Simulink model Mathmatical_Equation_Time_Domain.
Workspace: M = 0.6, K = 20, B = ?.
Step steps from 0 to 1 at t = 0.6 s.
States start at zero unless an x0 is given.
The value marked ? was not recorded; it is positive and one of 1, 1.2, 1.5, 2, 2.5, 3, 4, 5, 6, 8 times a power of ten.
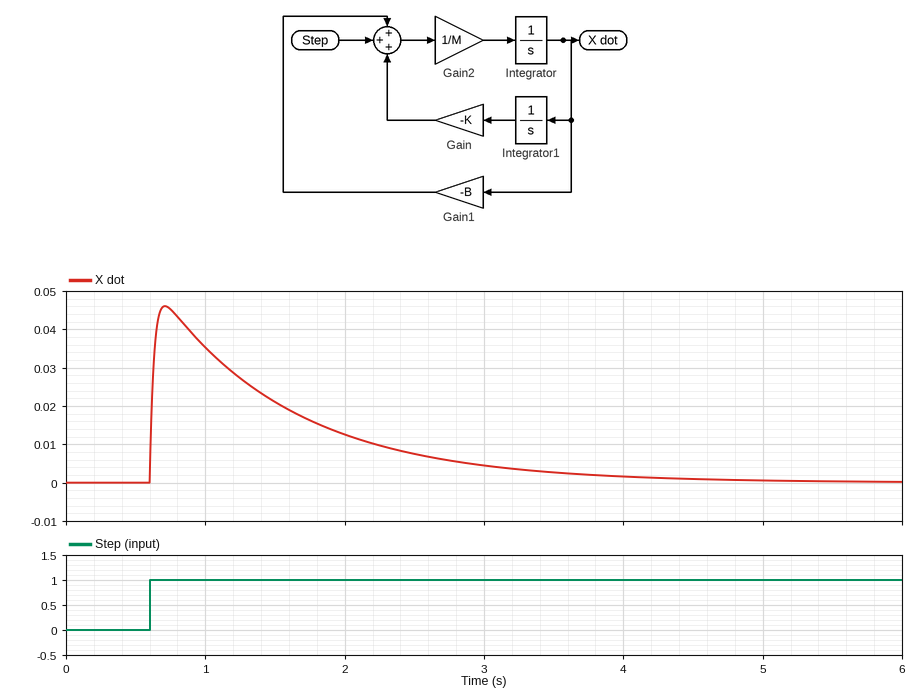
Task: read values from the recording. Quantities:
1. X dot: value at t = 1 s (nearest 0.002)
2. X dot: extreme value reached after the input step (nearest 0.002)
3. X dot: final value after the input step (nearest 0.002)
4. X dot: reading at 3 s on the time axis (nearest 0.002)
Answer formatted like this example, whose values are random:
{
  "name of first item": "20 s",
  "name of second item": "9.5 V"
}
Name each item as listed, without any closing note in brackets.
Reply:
{
  "X dot: value at t = 1 s": "0.036",
  "X dot: extreme value reached after the input step": "0.046",
  "X dot: final value after the input step": "0.000",
  "X dot: reading at 3 s on the time axis": "0.004"
}
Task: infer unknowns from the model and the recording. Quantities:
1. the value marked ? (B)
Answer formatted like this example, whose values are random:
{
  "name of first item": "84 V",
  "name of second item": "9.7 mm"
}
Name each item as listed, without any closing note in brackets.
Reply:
{
  "the value marked ?": "20"
}
